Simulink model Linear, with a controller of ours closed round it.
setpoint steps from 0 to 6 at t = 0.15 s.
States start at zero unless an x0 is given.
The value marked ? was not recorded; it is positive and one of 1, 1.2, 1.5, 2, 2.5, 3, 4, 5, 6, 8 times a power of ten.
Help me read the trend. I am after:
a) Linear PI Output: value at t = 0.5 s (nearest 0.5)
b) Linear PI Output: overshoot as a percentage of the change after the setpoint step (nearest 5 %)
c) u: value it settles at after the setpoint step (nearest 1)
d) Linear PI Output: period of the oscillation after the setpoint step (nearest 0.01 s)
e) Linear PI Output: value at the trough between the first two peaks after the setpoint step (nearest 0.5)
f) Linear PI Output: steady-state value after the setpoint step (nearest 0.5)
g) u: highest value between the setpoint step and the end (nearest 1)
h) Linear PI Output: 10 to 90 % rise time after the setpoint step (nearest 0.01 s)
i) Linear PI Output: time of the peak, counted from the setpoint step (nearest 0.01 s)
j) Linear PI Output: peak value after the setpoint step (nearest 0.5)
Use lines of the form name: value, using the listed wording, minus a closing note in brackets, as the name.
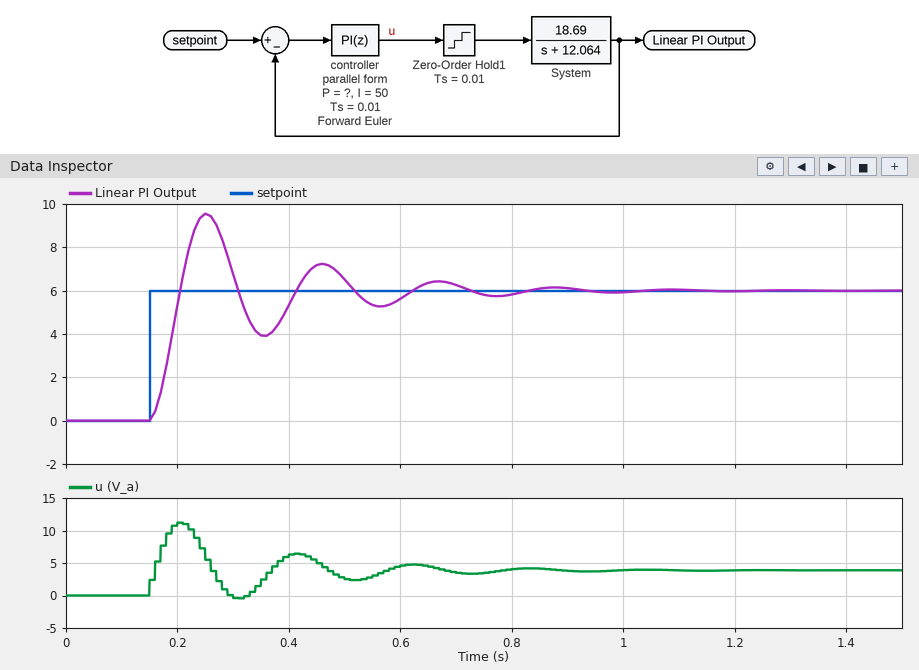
Linear PI Output: value at t = 0.5 s: 6.5
Linear PI Output: overshoot as a percentage of the change after the setpoint step: 60 %
u: value it settles at after the setpoint step: 4
Linear PI Output: period of the oscillation after the setpoint step: 0.21 s
Linear PI Output: value at the trough between the first two peaks after the setpoint step: 4.0
Linear PI Output: steady-state value after the setpoint step: 6.0
u: highest value between the setpoint step and the end: 11
Linear PI Output: 10 to 90 % rise time after the setpoint step: 0.04 s
Linear PI Output: time of the peak, counted from the setpoint step: 0.10 s
Linear PI Output: peak value after the setpoint step: 9.5
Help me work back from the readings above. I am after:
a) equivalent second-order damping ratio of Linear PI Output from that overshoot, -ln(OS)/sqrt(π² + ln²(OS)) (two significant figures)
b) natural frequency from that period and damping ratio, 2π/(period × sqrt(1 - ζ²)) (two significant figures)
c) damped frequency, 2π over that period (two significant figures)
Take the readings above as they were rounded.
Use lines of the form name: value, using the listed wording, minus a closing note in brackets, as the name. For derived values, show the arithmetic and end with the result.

equivalent second-order damping ratio of Linear PI Output from that overshoot, -ln(OS)/sqrt(π² + ln²(OS)): ln(0.6) = -0.511; 0.511 / sqrt(9.870 + 0.261) = 0.16
natural frequency from that period and damping ratio, 2π/(period × sqrt(1 - ζ²)): 2π / (0.21 × sqrt(1 - 0.16²)) = 30 rad/s
damped frequency, 2π over that period: 2π / 0.21 = 30 rad/s
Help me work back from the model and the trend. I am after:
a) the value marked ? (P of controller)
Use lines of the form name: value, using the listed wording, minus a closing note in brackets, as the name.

the value marked ?: 0.4
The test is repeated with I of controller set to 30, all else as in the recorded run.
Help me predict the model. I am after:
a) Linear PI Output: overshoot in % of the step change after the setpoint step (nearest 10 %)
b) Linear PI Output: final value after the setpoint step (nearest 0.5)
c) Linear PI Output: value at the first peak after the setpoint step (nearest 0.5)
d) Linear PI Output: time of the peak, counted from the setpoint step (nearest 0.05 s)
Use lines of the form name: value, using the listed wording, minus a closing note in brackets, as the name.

Linear PI Output: overshoot in % of the step change after the setpoint step: 40 %
Linear PI Output: final value after the setpoint step: 6.0
Linear PI Output: value at the first peak after the setpoint step: 8.5
Linear PI Output: time of the peak, counted from the setpoint step: 0.15 s
